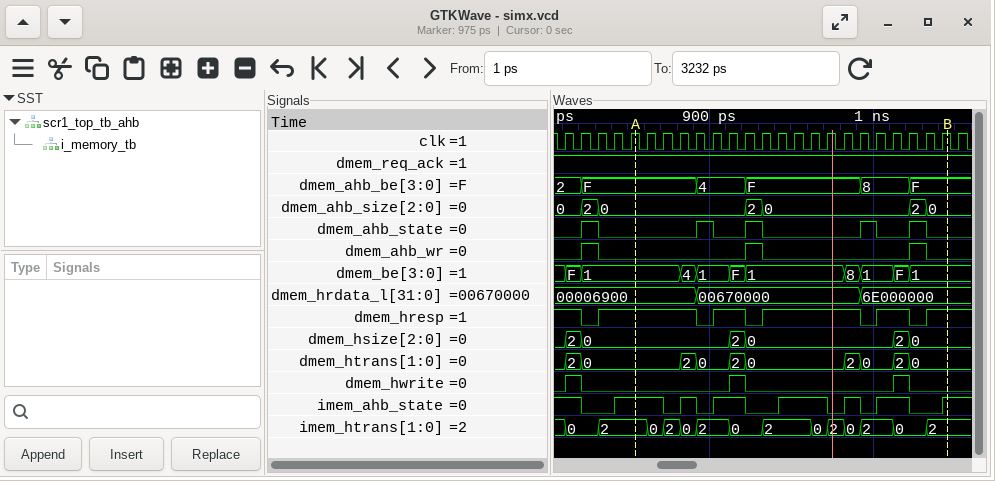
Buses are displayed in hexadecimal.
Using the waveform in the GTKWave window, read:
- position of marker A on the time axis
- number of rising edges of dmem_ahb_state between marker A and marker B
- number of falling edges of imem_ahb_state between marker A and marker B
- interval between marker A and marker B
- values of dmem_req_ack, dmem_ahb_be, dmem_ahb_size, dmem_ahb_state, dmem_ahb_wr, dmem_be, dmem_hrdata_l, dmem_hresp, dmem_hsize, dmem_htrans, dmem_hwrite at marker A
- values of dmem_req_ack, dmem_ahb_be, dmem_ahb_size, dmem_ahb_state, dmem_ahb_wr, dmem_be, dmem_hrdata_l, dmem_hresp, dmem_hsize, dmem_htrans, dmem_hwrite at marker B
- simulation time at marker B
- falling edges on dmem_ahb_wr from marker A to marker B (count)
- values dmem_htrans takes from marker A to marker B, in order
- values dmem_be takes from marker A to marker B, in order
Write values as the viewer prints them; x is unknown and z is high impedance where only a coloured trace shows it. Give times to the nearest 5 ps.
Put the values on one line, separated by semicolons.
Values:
855 ps; 4; 6; 190 ps; dmem_req_ack=1, dmem_ahb_be=F, dmem_ahb_size=0, dmem_ahb_state=0, dmem_ahb_wr=0, dmem_be=1, dmem_hrdata_l=00006900, dmem_hresp=1, dmem_hsize=0, dmem_htrans=0, dmem_hwrite=0; dmem_req_ack=1, dmem_ahb_be=F, dmem_ahb_size=0, dmem_ahb_state=0, dmem_ahb_wr=0, dmem_be=1, dmem_hrdata_l=6E000000, dmem_hresp=1, dmem_hsize=0, dmem_htrans=0, dmem_hwrite=0; 1045 ps; 2; 0, 2, 0, 2, 0, 2, 0, 2, 0; 1, 4, 1, F, 1, 8, 1, F, 1
